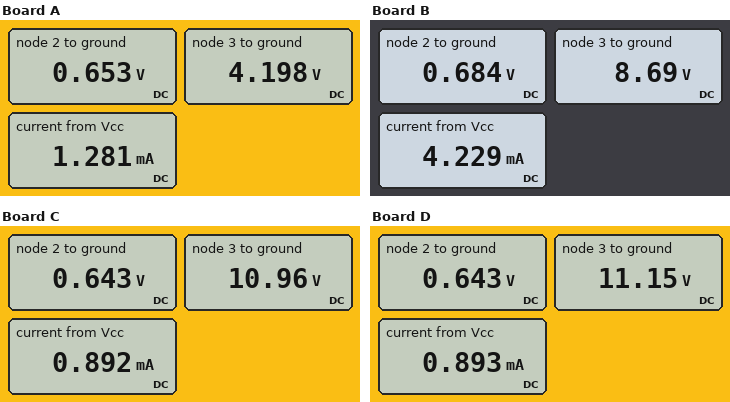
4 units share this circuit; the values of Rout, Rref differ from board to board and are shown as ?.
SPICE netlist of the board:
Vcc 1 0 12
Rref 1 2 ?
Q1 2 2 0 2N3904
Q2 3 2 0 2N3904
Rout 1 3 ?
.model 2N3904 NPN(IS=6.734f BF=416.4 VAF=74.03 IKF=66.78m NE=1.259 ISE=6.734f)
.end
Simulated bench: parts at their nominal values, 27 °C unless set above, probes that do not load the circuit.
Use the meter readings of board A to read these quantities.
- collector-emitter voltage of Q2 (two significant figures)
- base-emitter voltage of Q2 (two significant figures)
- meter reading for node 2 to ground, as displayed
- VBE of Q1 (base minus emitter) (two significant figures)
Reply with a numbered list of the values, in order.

1. 4.2 V
2. 650 mV
3. 0.653 V
4. 650 mV
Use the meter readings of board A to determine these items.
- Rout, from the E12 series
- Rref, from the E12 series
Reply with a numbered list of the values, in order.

1. 12 kΩ
2. 18 kΩ
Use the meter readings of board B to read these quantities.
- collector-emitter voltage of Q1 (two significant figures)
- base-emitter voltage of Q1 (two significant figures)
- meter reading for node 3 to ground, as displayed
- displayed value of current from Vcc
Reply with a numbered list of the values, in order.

1. 680 mV
2. 680 mV
3. 8.69 V
4. 4.229 mA
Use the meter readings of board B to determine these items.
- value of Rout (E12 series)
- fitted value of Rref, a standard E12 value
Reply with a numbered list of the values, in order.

1. 1.5 kΩ
2. 5.6 kΩ
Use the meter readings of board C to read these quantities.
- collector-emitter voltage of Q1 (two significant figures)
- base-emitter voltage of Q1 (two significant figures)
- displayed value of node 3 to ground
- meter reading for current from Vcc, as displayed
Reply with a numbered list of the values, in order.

1. 640 mV
2. 640 mV
3. 10.96 V
4. 0.892 mA
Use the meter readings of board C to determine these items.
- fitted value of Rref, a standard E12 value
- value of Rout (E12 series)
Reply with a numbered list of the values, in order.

1. 27 kΩ
2. 2.2 kΩ
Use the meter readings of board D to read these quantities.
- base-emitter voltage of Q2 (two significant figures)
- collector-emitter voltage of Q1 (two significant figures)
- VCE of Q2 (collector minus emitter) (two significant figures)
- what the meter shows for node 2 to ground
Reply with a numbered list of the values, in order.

1. 640 mV
2. 640 mV
3. 11 V
4. 0.643 V
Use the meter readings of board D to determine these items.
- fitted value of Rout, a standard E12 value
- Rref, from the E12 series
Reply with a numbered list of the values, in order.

1. 1.8 kΩ
2. 27 kΩ
